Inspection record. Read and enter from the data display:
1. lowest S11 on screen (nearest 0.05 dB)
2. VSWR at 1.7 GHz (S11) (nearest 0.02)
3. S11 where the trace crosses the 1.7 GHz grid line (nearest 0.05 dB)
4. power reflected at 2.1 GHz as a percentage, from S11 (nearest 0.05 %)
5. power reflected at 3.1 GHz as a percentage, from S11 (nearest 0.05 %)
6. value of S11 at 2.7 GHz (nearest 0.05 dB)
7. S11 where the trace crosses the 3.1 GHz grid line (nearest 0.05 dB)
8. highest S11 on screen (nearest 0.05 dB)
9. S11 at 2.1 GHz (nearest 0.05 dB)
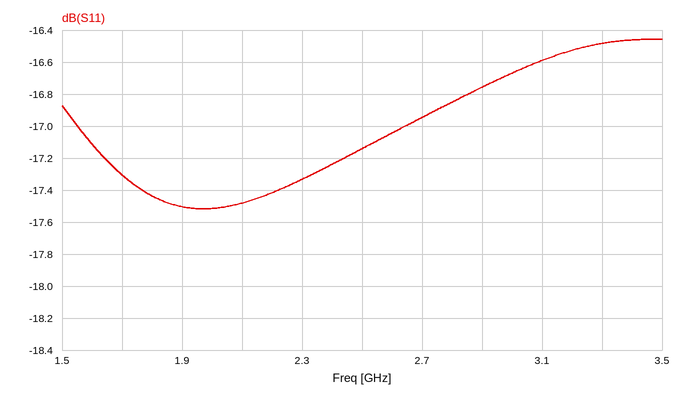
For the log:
-17.50 dB
1.32
-17.30 dB
1.80 %
2.20 %
-16.95 dB
-16.60 dB
-16.45 dB
-17.50 dB
